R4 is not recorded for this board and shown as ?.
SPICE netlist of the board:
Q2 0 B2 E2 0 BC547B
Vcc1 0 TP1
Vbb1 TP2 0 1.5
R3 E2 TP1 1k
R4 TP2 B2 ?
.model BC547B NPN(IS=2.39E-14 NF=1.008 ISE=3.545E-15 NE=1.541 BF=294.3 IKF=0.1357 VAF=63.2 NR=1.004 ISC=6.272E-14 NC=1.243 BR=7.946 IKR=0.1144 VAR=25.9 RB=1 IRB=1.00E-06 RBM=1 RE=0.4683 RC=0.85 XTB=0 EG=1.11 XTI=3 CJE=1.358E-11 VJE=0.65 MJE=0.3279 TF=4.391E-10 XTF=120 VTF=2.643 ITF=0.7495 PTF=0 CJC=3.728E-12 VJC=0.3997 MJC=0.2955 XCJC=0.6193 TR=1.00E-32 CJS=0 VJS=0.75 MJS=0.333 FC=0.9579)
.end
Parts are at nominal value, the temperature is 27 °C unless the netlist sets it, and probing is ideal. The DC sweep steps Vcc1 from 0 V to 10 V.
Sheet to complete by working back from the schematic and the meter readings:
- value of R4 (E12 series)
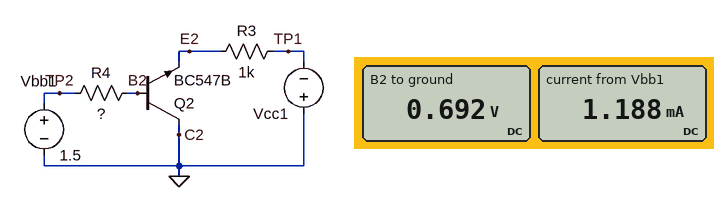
680 Ω
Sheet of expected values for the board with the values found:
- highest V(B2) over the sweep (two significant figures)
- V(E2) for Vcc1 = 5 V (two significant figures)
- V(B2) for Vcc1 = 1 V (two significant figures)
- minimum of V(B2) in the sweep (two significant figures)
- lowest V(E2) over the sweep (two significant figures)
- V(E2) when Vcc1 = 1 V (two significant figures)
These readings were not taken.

690 mV
-23 mV
690 mV
680 mV
-39 mV
-6.4 mV
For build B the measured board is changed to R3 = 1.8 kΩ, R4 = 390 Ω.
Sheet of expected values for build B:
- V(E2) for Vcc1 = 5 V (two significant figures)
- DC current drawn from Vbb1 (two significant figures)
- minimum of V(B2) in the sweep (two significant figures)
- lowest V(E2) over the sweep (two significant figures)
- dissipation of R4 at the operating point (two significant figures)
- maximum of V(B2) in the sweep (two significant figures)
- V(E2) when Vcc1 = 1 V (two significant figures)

-10 mV
2.0 mA
700 mV
-19 mV
1.6 mW
710 mV
-2.9 mV
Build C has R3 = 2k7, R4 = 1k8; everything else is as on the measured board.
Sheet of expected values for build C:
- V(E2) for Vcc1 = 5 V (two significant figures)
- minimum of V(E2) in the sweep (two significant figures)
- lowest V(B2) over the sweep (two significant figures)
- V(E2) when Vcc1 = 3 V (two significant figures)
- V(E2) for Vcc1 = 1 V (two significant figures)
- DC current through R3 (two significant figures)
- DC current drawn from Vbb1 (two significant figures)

-18 mV
-29 mV
660 mV
-12 mV
-5.8 mV
800 nA
460 µA
